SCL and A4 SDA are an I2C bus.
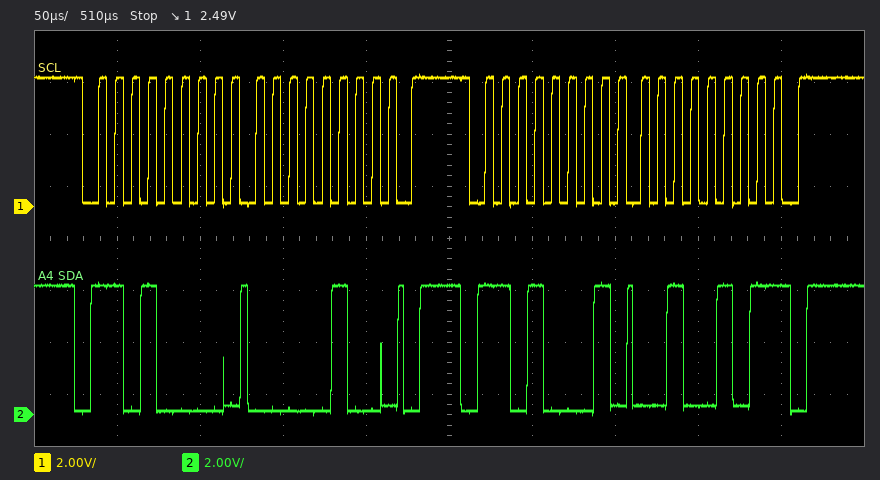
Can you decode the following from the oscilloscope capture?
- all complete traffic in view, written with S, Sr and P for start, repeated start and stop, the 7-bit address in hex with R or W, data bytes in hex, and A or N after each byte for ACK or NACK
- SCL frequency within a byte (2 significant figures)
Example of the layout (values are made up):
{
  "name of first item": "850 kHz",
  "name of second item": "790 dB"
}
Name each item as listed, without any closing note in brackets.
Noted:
{
  "all complete traffic in view, written with S, Sr and P for start, repeated start and stop, the 7-bit address in hex with R or W, data bytes in hex, and A or N after each byte for ACK or NACK": "S 68W A 04 A P S 68R A 25 N P",
  "SCL frequency within a byte": "100 kHz"
}
